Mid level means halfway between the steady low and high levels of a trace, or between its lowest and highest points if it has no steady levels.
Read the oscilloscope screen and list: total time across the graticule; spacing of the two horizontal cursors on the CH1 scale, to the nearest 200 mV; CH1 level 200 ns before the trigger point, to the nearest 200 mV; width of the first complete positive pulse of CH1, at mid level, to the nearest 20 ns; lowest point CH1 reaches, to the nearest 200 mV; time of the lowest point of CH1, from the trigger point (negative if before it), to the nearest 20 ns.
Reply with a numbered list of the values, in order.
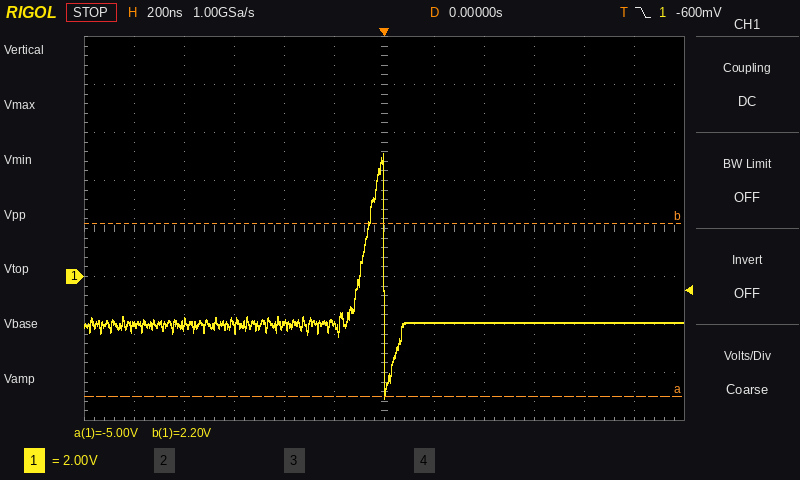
1. 2.4 µs
2. 7.2 V
3. -2.0 V
4. 100 ns
5. -5.0 V
6. 0 ns
